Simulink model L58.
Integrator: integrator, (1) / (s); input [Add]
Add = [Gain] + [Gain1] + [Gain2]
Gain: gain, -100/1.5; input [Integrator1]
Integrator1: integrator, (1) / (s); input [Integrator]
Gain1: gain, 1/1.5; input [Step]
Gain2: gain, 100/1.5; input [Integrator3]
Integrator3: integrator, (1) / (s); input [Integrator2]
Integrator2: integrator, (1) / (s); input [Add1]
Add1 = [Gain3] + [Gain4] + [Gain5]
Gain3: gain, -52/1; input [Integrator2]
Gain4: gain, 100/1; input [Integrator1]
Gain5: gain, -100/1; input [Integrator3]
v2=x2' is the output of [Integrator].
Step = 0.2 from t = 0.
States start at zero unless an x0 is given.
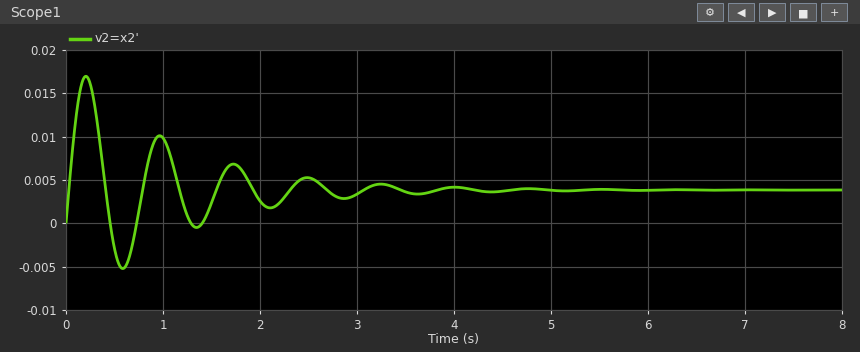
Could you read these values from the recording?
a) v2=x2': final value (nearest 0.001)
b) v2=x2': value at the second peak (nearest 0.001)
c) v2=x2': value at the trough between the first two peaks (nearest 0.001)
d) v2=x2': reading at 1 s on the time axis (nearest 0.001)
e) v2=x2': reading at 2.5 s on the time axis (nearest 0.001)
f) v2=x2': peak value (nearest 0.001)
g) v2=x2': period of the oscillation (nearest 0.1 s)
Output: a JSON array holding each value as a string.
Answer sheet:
["0.004", "0.010", "-0.005", "0.010", "0.005", "0.017", "0.8 s"]
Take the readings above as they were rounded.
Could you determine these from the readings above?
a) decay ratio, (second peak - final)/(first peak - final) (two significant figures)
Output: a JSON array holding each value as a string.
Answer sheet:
["0.46"]
